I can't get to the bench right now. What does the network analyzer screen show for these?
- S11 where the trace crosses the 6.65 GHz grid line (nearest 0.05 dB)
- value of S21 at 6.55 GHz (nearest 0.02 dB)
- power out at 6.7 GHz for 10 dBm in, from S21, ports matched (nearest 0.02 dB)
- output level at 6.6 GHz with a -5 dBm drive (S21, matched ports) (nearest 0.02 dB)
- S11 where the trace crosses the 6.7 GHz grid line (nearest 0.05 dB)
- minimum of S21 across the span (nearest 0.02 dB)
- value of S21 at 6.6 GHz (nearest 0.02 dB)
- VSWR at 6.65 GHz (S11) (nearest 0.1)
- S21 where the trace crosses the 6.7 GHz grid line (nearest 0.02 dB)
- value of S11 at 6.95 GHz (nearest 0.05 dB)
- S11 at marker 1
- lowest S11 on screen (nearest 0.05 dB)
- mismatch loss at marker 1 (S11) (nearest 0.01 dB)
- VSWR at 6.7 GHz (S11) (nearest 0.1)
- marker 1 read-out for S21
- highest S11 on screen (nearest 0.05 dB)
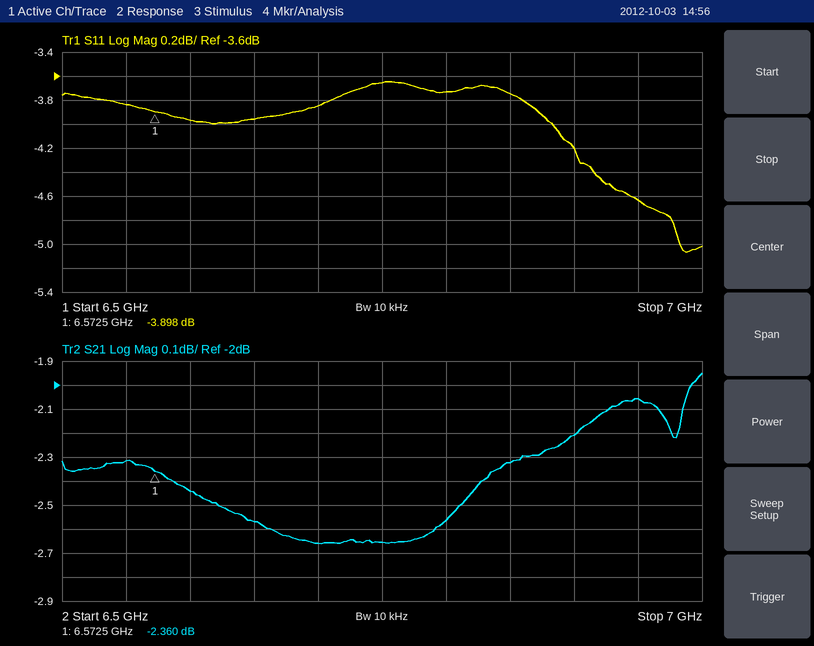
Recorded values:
-3.95 dB
-2.32 dB
7.34 dBm
-7.44 dBm
-3.85 dB
-2.66 dB
-2.44 dB
4.5
-2.66 dB
-4.65 dB
-3.898 dB
-5.05 dB
2.27 dB
4.6
-2.360 dB
-3.65 dB
